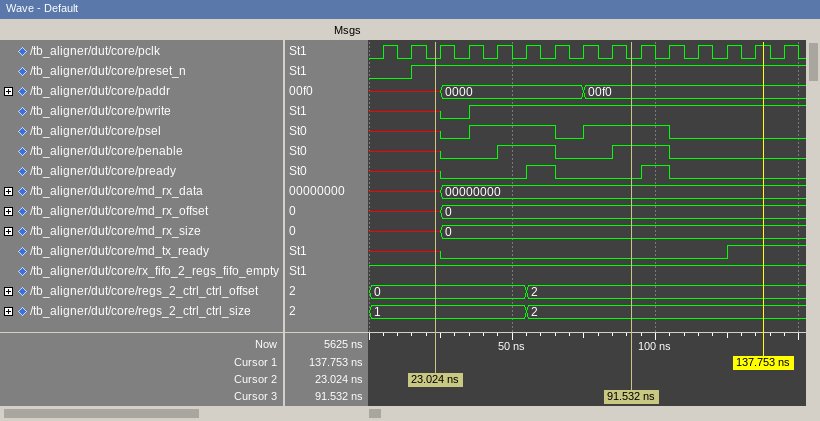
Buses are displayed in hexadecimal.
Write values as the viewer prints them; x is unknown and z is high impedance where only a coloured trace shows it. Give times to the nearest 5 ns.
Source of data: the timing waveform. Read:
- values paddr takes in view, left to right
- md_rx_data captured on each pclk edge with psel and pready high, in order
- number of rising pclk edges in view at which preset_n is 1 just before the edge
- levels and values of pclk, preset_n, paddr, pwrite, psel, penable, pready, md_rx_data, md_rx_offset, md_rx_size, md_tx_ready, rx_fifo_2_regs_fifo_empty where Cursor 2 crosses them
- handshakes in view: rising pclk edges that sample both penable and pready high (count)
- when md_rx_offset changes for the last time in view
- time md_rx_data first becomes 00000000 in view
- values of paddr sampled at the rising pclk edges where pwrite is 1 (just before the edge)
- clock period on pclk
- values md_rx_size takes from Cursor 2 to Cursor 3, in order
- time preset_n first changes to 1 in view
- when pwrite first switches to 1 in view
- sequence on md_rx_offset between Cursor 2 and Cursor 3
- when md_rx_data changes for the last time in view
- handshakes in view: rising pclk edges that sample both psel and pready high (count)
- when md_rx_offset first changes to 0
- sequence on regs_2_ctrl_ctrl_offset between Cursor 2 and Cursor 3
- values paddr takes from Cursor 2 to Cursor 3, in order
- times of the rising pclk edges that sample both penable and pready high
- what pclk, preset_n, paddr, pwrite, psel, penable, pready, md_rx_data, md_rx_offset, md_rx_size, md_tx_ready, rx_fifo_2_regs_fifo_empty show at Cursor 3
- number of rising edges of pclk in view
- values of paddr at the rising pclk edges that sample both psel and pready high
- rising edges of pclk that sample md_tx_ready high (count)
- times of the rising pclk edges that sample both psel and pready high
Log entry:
x, 0000, 00f0
00000000, 00000000
13
pclk=0, preset_n=1, paddr=x, pwrite=x, psel=x, penable=x, pready=x, md_rx_data=x, md_rx_offset=x, md_rx_size=x, md_tx_ready=x, rx_fifo_2_regs_fifo_empty=1
2
25 ns
25 ns
0000, 0000, 0000, 0000, 00f0, 00f0, 00f0, 00f0, 00f0, 00f0, 00f0
10 ns
x, 0
15 ns
35 ns
x, 0
25 ns
2
25 ns
0, 2
x, 0000, 00f0
65 ns, 105 ns
pclk=0, preset_n=1, paddr=00f0, pwrite=1, psel=1, penable=1, pready=0, md_rx_data=00000000, md_rx_offset=0, md_rx_size=0, md_tx_ready=0, rx_fifo_2_regs_fifo_empty=1
15
0000, 00f0
2
65 ns, 105 ns
